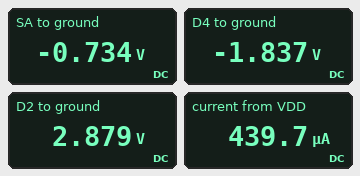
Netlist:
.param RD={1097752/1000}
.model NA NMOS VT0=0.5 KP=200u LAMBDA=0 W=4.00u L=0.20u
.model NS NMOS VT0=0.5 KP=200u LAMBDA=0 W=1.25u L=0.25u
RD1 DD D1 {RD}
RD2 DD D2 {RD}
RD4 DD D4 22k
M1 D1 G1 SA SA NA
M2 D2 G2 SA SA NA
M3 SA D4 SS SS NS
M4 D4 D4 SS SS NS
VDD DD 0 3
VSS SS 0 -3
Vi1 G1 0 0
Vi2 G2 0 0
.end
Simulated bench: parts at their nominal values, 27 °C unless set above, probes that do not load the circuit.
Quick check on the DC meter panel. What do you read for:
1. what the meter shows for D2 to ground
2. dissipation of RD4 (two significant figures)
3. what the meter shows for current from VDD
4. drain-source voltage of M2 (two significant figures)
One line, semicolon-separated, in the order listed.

2.879 V; 1.1 mW; 439.7 µA; 3.6 V
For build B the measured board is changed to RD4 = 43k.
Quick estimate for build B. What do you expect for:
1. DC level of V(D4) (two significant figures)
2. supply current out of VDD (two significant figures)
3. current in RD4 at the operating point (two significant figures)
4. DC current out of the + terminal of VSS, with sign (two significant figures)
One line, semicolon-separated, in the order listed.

-2.0 V; 230 µA; 120 µA; -230 µA
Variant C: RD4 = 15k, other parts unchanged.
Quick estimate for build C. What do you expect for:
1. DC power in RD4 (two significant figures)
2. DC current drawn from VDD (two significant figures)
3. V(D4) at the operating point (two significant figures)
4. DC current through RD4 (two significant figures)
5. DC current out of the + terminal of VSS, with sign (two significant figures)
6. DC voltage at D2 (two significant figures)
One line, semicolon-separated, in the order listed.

1.5 mW; 630 µA; -1.7 V; 310 µA; -630 µA; 2.8 V
